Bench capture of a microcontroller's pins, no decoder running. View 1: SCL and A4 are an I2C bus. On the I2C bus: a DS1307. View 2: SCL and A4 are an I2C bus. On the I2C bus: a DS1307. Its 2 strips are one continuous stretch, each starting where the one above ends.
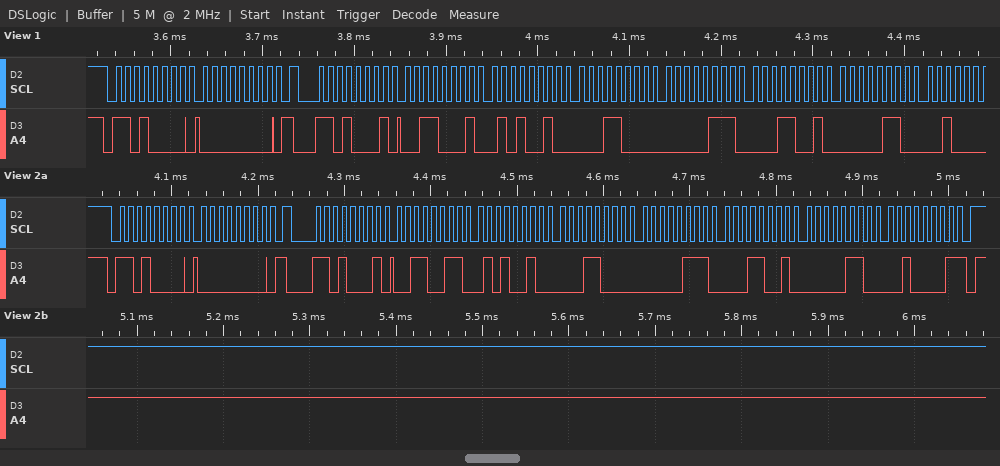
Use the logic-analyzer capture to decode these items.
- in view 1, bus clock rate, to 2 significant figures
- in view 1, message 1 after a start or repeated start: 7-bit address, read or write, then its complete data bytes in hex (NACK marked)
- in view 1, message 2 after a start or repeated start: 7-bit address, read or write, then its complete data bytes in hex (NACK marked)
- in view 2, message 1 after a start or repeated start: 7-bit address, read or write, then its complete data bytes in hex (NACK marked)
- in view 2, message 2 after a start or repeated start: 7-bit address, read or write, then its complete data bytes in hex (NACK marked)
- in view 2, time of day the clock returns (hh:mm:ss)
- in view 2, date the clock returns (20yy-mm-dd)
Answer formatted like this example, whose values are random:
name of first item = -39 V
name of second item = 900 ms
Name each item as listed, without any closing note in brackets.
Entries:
in view 1, bus clock rate, to 2 significant figures = 100 kHz
in view 1, message 1 after a start or repeated start: 7-bit address, read or write, then its complete data bytes in hex = 0x68 write: 00
in view 1, message 2 after a start or repeated start: 7-bit address, read or write, then its complete data bytes in hex = 0x68 read: 31 52 18 07 19 06
in view 2, message 1 after a start or repeated start: 7-bit address, read or write, then its complete data bytes in hex = 0x68 write: 00
in view 2, message 2 after a start or repeated start: 7-bit address, read or write, then its complete data bytes in hex = 0x68 read: 33 52 18 07 19 06 21 NACK
in view 2, time of day the clock returns = 18:52:33
in view 2, date the clock returns = 2021-06-19
